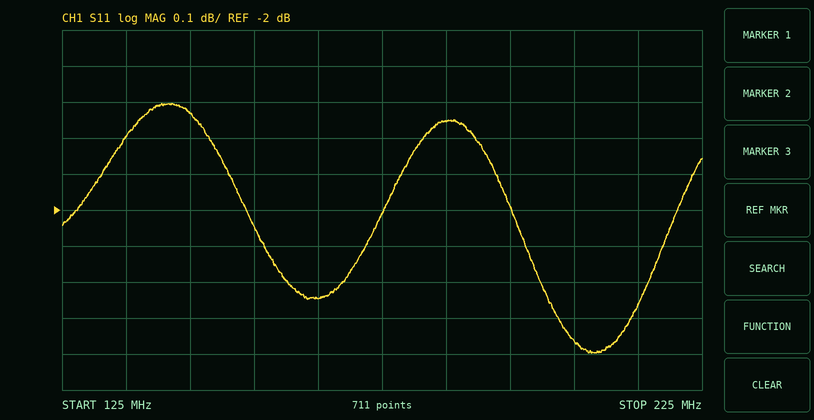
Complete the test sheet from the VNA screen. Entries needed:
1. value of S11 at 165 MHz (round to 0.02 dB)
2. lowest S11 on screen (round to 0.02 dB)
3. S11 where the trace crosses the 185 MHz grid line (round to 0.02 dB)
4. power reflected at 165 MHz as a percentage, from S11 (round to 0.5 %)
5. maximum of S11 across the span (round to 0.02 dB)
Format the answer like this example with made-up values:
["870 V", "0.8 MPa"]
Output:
["-2.24 dB", "-2.40 dB", "-1.76 dB", "59.5 %", "-1.70 dB"]
